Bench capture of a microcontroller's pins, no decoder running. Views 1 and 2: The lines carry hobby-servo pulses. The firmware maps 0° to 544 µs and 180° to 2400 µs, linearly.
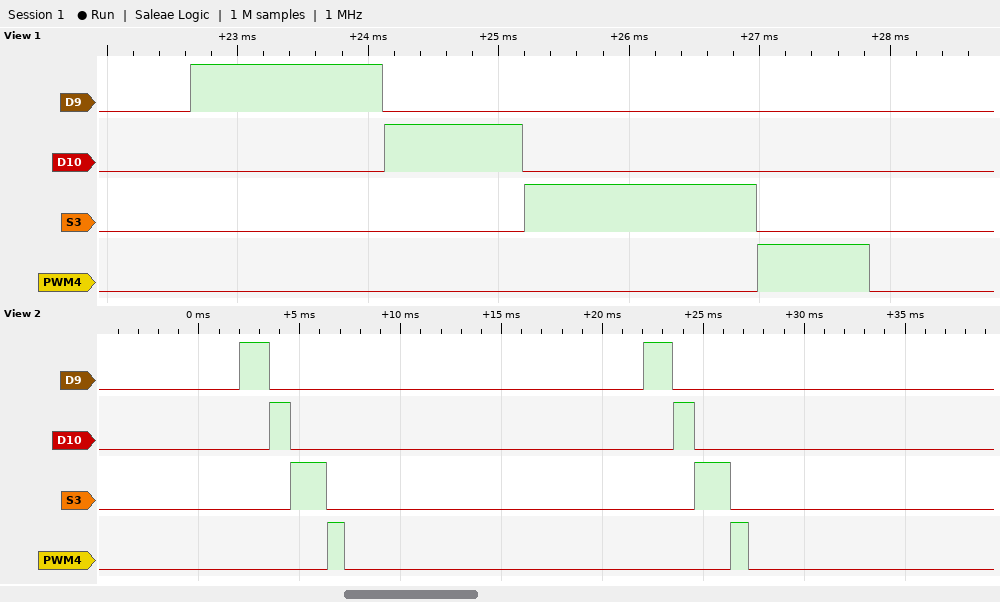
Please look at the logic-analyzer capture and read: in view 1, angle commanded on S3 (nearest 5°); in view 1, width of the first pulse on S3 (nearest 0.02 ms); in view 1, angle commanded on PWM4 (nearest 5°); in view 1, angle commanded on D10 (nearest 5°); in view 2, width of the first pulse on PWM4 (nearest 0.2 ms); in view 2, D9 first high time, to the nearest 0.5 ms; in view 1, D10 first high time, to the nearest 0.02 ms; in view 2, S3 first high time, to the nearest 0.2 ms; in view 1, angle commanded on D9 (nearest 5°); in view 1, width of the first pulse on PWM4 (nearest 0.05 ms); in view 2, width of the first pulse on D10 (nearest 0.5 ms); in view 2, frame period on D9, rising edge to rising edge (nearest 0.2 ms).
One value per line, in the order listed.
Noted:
120°
1.78 ms
30°
50°
0.8 ms
1.5 ms
1.06 ms
1.8 ms
90°
0.85 ms
1.0 ms
20.0 ms
